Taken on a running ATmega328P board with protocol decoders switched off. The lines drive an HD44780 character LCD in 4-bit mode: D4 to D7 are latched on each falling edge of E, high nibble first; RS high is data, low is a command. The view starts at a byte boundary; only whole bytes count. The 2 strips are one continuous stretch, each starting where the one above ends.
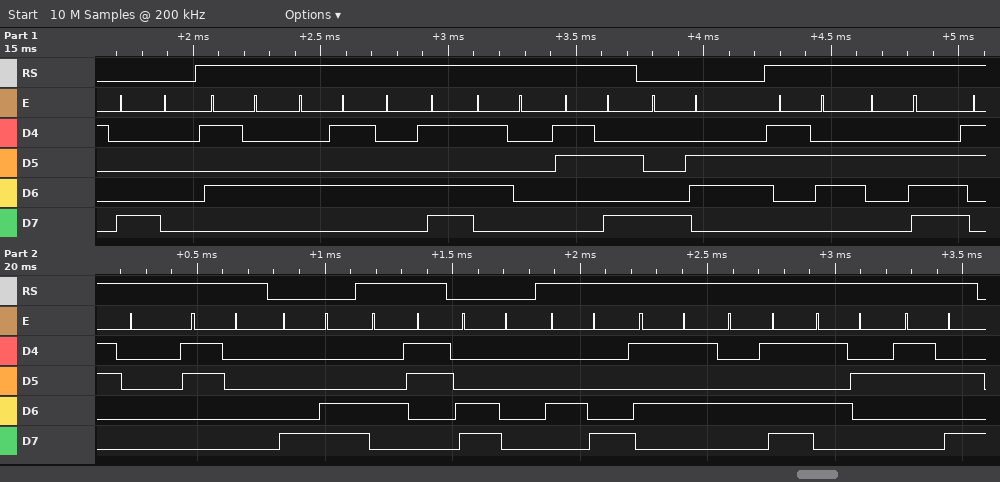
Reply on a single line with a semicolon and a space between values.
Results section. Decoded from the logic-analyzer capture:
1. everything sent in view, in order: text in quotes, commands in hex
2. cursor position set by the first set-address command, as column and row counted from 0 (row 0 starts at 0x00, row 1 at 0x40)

0x80 "TEMP:" 0x86 "6.00" 0x8C "C" 0xC0 "HUMR:"; column 0, row 0
